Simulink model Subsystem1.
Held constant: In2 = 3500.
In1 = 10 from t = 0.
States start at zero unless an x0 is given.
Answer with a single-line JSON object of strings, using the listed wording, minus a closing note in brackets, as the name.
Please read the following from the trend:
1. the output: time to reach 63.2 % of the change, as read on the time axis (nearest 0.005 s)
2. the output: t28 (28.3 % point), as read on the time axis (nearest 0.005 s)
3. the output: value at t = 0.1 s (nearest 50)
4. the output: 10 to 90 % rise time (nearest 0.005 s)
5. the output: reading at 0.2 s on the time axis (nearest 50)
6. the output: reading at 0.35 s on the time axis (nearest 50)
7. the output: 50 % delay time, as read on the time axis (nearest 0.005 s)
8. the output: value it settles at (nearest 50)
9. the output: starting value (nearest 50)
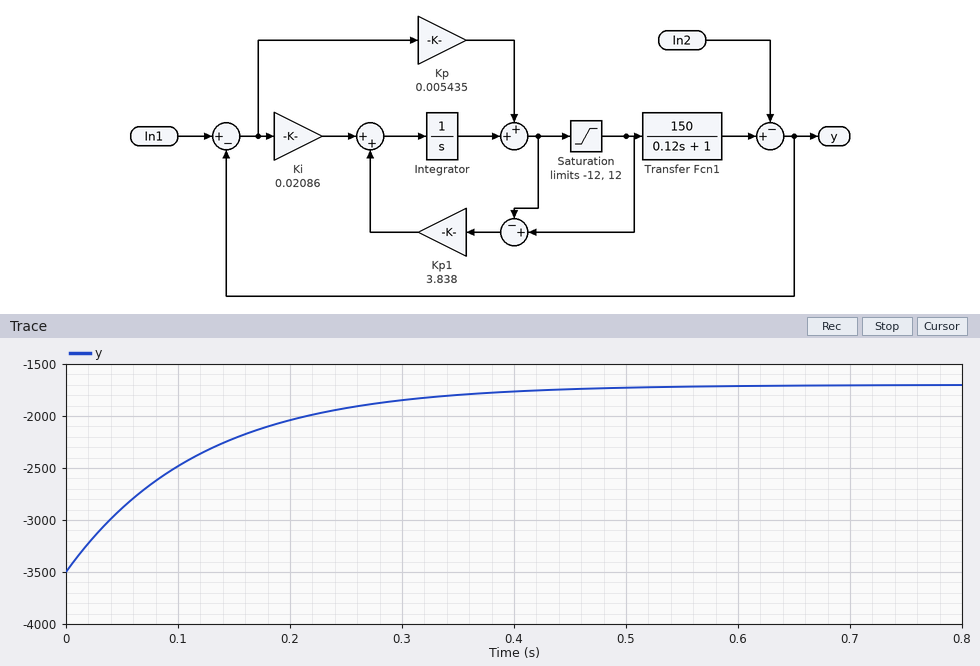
{"the output: time to reach 63.2 % of the change, as read on the time axis": "0.120 s", "the output: t28 (28.3 % point), as read on the time axis": "0.040 s", "the output: value at t = 0.1 s": "-2500", "the output: 10 to 90 % rise time": "0.265 s", "the output: reading at 0.2 s on the time axis": "-2050", "the output: reading at 0.35 s on the time axis": "-1800", "the output: 50 % delay time, as read on the time axis": "0.085 s", "the output: value it settles at": "-1700", "the output: starting value": "-3500"}
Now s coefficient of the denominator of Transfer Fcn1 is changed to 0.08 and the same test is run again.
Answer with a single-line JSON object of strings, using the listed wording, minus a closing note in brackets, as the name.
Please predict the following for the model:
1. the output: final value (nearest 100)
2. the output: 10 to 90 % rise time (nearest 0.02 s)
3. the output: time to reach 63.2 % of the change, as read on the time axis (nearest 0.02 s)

{"the output: final value": "-1700", "the output: 10 to 90 % rise time": "0.18 s", "the output: time to reach 63.2 % of the change, as read on the time axis": "0.08 s"}
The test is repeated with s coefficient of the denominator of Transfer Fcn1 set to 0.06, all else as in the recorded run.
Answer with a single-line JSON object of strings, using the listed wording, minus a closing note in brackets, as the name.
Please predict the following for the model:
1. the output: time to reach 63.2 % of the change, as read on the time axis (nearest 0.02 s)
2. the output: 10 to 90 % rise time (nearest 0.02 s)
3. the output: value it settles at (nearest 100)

{"the output: time to reach 63.2 % of the change, as read on the time axis": "0.06 s", "the output: 10 to 90 % rise time": "0.14 s", "the output: value it settles at": "-1700"}
